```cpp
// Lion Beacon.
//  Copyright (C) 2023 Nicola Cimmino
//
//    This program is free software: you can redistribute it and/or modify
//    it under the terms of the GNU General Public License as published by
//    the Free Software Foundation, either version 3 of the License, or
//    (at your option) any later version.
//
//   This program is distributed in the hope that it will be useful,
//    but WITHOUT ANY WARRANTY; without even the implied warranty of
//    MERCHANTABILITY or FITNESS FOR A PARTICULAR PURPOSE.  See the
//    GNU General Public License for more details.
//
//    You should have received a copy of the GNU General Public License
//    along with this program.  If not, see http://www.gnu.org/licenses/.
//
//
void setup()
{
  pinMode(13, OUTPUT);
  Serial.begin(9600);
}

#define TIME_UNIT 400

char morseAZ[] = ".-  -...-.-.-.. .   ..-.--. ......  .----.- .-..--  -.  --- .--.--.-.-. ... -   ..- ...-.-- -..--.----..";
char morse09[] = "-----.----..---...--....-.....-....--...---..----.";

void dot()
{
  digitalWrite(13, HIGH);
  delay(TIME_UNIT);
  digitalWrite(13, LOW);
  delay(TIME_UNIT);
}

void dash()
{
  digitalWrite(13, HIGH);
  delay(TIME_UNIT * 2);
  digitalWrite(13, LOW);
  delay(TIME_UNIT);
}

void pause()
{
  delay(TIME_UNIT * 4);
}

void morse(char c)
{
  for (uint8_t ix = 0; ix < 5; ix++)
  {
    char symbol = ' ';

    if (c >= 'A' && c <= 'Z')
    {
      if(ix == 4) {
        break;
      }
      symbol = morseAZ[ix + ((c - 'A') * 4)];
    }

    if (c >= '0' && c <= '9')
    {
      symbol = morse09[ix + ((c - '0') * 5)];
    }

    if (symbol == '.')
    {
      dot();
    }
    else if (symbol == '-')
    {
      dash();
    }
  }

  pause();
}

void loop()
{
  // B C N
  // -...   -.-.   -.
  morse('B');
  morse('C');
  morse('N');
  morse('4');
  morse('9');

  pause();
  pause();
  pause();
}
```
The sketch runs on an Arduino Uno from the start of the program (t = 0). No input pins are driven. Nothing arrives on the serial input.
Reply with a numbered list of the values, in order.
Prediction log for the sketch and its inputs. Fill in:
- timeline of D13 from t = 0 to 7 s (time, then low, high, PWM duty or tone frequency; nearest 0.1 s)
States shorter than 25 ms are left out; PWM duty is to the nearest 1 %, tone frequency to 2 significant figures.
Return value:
1. 0 s high; 0.8 s low; 1.2 s high; 1.6 s low; 2 s high; 2.4 s low; 2.8 s high; 3.2 s low; 5.2 s high; 6 s low; 6.4 s high; 6.8 s low
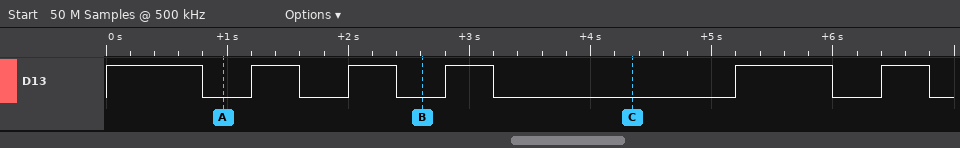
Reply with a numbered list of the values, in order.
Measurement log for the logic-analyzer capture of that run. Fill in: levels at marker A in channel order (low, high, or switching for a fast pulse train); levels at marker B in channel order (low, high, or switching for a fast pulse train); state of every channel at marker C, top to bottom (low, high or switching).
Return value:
1. D13 low
2. D13 low
3. D13 low
